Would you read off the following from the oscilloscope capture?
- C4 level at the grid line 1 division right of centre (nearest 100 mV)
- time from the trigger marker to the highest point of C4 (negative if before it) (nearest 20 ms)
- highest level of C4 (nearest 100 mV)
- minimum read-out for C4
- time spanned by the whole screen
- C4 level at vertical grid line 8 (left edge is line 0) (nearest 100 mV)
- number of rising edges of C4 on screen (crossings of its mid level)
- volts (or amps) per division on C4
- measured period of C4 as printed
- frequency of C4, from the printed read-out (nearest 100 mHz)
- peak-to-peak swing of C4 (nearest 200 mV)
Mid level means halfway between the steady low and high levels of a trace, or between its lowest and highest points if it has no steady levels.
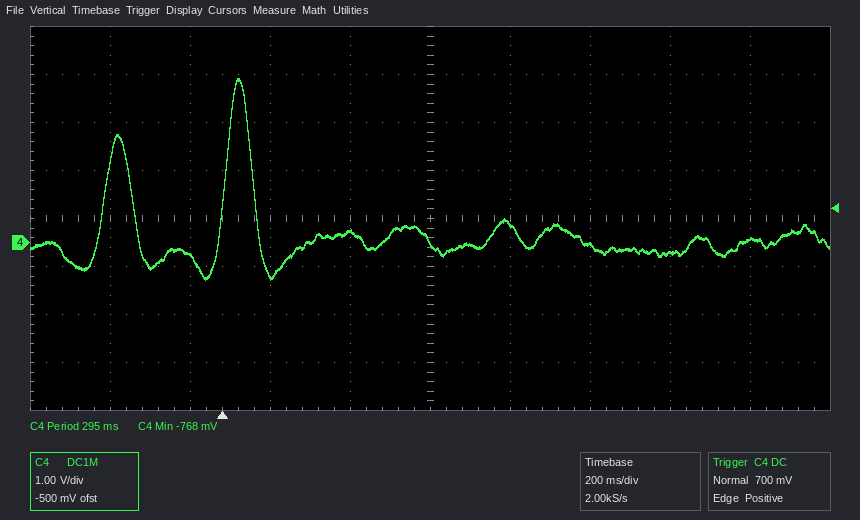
400 mV
+40 ms
3.4 V
-768 mV
2 s
-200 mV
2
1 V
295 ms
3.4 Hz
4.2 V
